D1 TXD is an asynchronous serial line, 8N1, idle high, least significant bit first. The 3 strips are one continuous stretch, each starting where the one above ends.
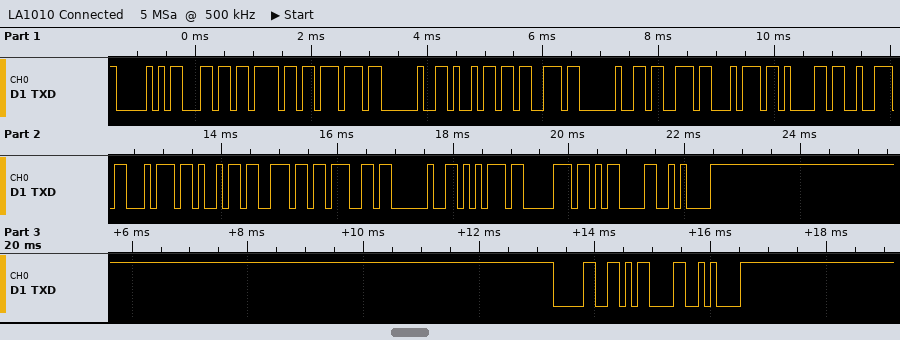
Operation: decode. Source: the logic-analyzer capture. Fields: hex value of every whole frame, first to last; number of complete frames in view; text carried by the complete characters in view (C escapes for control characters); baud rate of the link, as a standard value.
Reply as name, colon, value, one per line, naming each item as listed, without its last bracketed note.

hex value of every whole frame, first to last: 50 6C 6F 77 20 69 73 20 73 74 61 72 74 69 6E 67 20 75 70 0D 0A 30 0D 0A
number of complete frames in view: 24
text carried by the complete characters in view: "Plow is starting up\r\n0\r\n"
baud rate of the link, as a standard value: 9600 baud
